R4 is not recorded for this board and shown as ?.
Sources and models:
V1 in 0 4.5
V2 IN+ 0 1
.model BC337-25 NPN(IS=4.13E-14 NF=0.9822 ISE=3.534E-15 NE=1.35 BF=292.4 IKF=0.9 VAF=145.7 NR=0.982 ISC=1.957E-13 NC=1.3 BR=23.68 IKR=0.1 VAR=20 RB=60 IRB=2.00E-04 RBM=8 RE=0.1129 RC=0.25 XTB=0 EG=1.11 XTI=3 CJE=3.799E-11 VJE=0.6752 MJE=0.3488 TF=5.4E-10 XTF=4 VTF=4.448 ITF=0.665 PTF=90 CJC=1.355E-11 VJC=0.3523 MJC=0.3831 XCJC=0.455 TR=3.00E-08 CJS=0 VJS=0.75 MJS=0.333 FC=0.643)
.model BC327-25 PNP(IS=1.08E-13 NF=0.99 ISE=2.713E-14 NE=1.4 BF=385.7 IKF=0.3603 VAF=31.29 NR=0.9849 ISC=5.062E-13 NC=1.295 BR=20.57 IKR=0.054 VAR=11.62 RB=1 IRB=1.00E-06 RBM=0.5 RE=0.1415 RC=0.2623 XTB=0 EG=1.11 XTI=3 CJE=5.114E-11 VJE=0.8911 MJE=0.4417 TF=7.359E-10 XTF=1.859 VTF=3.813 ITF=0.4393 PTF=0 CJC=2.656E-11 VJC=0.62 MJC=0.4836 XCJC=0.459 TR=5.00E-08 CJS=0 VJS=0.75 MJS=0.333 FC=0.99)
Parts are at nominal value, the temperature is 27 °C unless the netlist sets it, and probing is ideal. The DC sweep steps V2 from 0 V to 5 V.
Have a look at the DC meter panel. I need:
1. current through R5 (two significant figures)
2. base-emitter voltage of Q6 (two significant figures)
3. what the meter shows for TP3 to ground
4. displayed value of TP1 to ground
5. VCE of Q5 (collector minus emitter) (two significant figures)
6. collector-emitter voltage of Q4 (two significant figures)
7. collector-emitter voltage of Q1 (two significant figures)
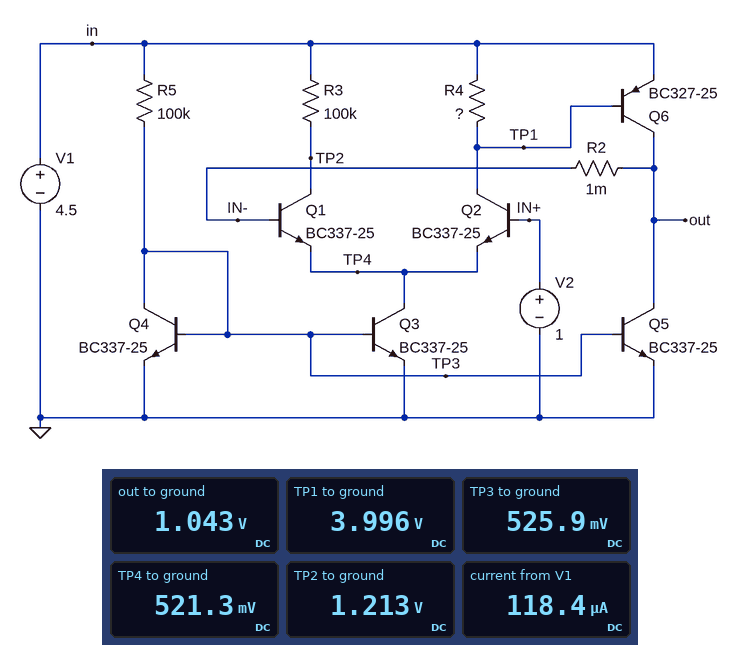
40 µA
-500 mV
525.9 mV
3.996 V
1.0 V
530 mV
690 mV
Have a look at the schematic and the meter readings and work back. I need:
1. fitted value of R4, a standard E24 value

82 kΩ
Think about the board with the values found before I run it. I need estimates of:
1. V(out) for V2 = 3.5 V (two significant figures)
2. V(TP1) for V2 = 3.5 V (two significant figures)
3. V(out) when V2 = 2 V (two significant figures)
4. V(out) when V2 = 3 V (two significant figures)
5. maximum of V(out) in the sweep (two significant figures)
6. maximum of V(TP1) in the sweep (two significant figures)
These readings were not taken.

3.6 V
4.0 V
2.1 V
3.1 V
4.5 V
4.5 V
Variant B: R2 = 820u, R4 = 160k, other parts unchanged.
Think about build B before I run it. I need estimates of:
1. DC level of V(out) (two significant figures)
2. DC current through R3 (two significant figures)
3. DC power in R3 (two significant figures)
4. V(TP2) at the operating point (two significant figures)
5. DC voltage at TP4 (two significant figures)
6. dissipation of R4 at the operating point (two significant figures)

1.1 V
36 µA
130 µW
910 mV
540 mV
1.6 µW
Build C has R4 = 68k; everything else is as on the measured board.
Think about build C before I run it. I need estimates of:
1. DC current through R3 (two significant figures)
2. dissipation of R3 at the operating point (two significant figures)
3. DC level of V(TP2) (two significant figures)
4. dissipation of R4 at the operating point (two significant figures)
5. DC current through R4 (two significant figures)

32 µA
100 µW
1.3 V
3.7 µW
7.4 µA
